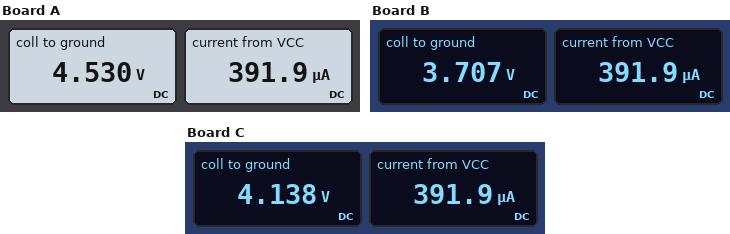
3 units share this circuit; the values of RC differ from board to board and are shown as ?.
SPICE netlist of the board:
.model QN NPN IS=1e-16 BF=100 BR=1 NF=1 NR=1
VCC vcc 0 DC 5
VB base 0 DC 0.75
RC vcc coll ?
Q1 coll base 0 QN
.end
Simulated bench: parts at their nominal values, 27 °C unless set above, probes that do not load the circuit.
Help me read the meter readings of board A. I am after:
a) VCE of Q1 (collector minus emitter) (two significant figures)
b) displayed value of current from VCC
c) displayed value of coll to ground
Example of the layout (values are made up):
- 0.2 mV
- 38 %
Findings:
- 4.5 V
- 391.9 µA
- 4.530 V
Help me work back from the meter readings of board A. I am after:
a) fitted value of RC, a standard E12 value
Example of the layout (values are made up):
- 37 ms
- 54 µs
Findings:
- 1.2 kΩ
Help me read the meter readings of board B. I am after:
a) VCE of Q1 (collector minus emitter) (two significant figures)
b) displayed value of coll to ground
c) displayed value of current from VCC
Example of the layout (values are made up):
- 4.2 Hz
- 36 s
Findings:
- 3.7 V
- 3.707 V
- 391.9 µA
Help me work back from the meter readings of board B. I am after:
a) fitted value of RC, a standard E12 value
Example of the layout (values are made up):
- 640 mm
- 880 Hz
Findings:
- 3.3 kΩ
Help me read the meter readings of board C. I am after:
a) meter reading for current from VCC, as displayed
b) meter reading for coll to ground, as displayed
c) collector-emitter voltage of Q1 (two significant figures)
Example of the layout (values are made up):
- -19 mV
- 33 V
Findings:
- 391.9 µA
- 4.138 V
- 4.1 V
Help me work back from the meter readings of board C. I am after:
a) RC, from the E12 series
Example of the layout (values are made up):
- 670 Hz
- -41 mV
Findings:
- 2.2 kΩ
